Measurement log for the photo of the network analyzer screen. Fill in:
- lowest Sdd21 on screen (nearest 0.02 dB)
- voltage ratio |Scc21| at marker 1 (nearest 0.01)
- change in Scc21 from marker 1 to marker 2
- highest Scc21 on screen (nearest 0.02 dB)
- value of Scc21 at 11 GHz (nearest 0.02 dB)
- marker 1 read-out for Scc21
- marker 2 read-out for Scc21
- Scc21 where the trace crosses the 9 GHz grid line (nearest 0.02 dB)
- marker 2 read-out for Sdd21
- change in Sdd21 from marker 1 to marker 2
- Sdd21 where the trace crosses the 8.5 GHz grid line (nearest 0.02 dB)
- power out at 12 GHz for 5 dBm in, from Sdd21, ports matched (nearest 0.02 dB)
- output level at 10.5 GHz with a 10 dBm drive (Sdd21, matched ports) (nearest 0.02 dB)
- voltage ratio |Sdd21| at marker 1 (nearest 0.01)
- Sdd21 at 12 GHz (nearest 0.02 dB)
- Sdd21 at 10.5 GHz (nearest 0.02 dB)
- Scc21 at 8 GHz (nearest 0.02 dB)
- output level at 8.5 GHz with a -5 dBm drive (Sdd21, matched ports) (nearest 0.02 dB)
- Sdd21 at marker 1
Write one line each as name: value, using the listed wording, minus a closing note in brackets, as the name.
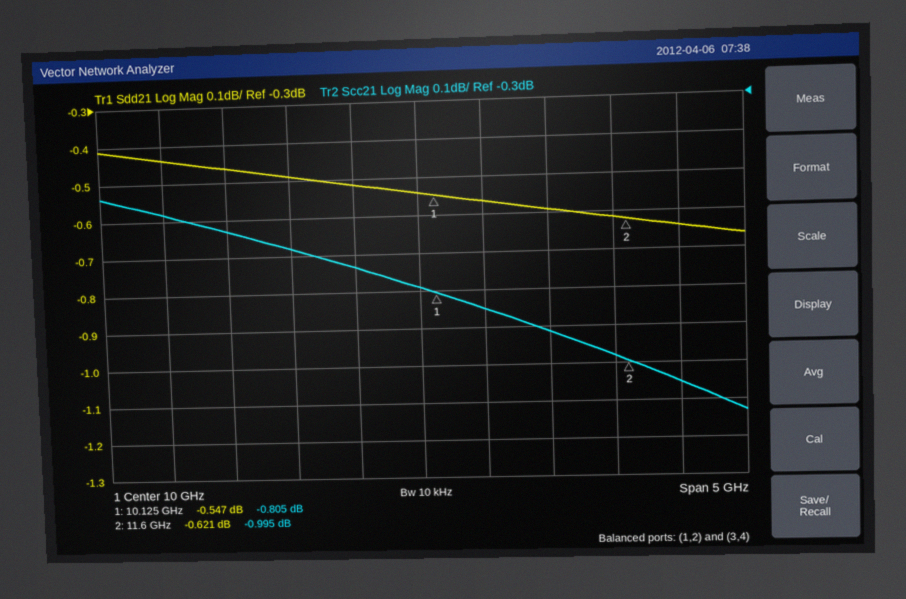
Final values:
lowest Sdd21 on screen: -0.66 dB
voltage ratio |Scc21| at marker 1: 0.91
change in Scc21 from marker 1 to marker 2: -0.190 dB
highest Scc21 on screen: -0.54 dB
value of Scc21 at 11 GHz: -0.92 dB
marker 1 read-out for Scc21: -0.805 dB
marker 2 read-out for Scc21: -0.995 dB
Scc21 where the trace crosses the 9 GHz grid line: -0.68 dB
marker 2 read-out for Sdd21: -0.621 dB
change in Sdd21 from marker 1 to marker 2: -0.074 dB
Sdd21 where the trace crosses the 8.5 GHz grid line: -0.46 dB
power out at 12 GHz for 5 dBm in, from Sdd21, ports matched: 4.36 dBm
output level at 10.5 GHz with a 10 dBm drive (Sdd21, matched ports): 9.44 dBm
voltage ratio |Sdd21| at marker 1: 0.94
Sdd21 at 12 GHz: -0.64 dB
Sdd21 at 10.5 GHz: -0.56 dB
Scc21 at 8 GHz: -0.58 dB
output level at 8.5 GHz with a -5 dBm drive (Sdd21, matched ports): -5.46 dBm
Sdd21 at marker 1: -0.547 dB
